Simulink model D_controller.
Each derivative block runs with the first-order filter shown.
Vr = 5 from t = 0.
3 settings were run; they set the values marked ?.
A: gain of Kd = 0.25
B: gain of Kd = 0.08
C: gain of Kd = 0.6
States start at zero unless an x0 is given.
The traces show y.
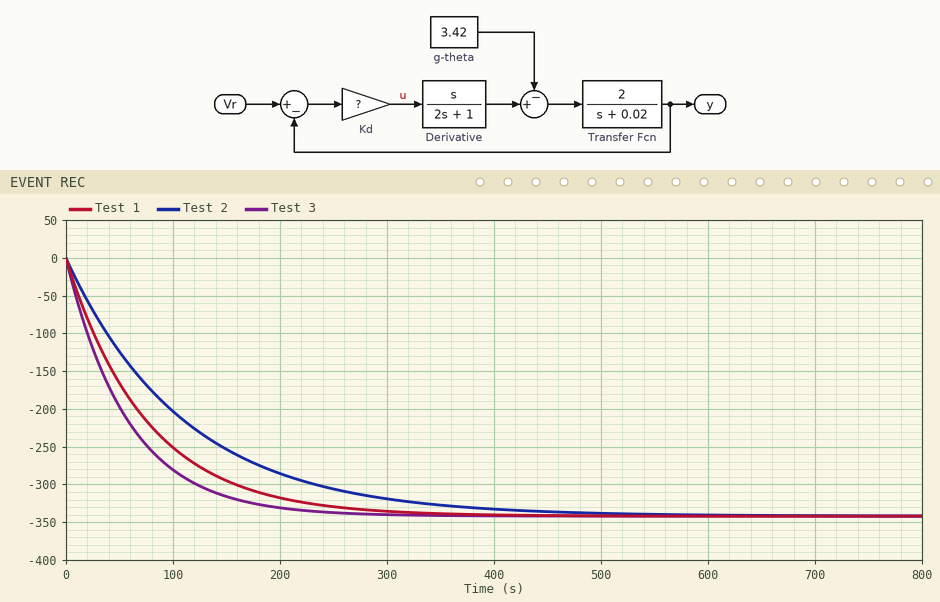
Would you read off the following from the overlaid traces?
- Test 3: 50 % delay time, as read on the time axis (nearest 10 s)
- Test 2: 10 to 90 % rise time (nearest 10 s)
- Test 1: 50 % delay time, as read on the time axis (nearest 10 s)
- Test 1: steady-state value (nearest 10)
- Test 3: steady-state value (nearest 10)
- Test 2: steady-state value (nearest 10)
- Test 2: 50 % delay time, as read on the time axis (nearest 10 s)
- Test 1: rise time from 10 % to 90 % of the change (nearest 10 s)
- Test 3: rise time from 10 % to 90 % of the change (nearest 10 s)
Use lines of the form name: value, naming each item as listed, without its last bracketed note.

Test 3: 50 % delay time, as read on the time axis: 40 s
Test 2: 10 to 90 % rise time: 240 s
Test 1: 50 % delay time, as read on the time axis: 50 s
Test 1: steady-state value: -340
Test 3: steady-state value: -340
Test 2: steady-state value: -340
Test 2: 50 % delay time, as read on the time axis: 80 s
Test 1: rise time from 10 % to 90 % of the change: 170 s
Test 3: rise time from 10 % to 90 % of the change: 130 s
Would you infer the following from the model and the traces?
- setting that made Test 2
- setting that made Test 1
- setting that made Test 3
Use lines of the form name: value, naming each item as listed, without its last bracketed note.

setting that made Test 2: C
setting that made Test 1: A
setting that made Test 3: B
